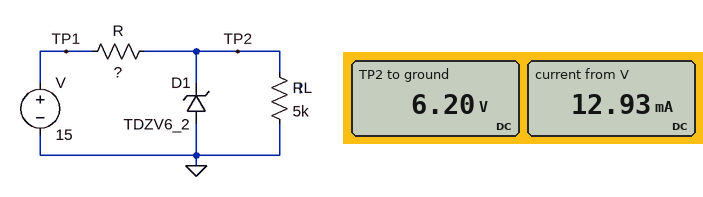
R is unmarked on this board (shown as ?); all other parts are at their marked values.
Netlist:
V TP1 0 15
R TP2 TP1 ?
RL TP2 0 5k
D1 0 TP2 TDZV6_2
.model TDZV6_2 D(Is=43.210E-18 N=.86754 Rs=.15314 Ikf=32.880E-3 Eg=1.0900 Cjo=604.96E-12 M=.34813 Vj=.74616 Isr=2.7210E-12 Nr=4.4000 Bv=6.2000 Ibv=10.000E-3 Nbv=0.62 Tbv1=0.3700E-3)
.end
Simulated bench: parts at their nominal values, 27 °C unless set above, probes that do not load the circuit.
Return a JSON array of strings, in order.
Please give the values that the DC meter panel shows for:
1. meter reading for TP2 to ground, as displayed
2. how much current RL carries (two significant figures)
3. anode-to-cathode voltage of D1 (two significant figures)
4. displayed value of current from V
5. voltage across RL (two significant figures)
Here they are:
["6.20 V", "1.2 mA", "-6.2 V", "12.93 mA", "6.2 V"]
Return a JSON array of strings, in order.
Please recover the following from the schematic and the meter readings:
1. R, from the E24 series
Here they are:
["680 Ω"]
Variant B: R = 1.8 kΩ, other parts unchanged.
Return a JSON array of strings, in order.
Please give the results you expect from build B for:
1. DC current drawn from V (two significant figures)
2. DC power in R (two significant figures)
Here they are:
["4.9 mA", "43 mW"]
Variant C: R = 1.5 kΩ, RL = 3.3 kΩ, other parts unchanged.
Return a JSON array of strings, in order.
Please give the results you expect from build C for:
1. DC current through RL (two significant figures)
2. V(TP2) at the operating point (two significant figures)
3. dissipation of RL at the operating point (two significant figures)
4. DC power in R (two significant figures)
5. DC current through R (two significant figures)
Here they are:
["1.9 mA", "6.2 V", "12 mW", "52 mW", "5.9 mA"]
